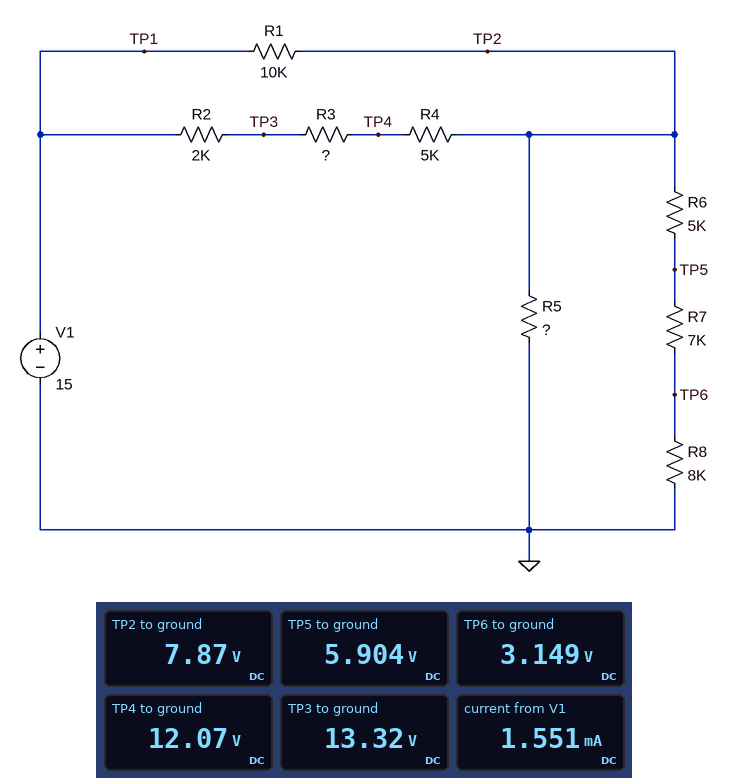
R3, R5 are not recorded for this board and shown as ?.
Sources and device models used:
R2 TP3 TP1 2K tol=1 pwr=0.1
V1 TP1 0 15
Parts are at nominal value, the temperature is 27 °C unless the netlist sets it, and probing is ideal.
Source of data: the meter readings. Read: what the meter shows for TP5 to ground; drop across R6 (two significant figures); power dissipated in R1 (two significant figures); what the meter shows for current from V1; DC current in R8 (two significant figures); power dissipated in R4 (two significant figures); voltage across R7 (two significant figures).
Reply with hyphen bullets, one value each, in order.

- 5.904 V
- 2.0 V
- 5.1 mW
- 1.551 mA
- 390 µA
- 3.5 mW
- 2.8 V
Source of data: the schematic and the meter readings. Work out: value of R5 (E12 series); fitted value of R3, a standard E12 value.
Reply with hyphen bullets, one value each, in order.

- 6.8 kΩ
- 1.5 kΩ
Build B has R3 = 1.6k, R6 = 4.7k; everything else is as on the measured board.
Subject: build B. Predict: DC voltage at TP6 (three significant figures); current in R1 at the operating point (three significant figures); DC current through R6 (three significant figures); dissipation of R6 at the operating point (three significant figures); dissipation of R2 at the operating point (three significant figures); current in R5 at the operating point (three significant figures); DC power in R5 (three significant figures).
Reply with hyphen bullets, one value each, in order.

- 3.18 V
- 717 µA
- 398 µA
- 743 µW
- 1.39 mW
- 1.15 mA
- 9.03 mW
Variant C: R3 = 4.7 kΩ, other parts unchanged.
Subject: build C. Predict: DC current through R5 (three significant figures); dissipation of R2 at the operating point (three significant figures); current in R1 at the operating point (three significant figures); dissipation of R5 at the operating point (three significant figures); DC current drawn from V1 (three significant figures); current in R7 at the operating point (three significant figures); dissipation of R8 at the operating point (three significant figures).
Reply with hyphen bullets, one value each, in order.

- 1.07 mA
- 872 µW
- 773 µA
- 7.78 mW
- 1.43 mA
- 364 µA
- 1.06 mW
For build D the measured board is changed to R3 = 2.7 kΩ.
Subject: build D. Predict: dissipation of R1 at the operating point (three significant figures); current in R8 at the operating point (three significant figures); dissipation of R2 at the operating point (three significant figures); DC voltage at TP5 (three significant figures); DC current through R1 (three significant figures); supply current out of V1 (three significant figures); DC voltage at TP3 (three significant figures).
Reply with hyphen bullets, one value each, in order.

- 5.46 mW
- 381 µA
- 1.16 mW
- 5.71 V
- 739 µA
- 1.50 mA
- 13.5 V
